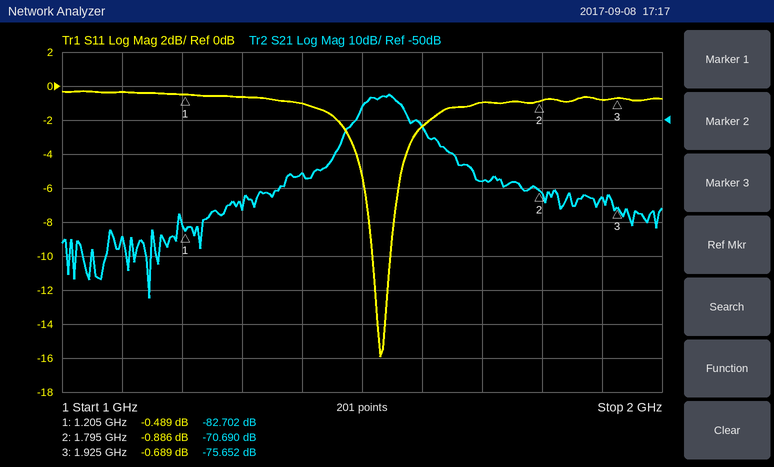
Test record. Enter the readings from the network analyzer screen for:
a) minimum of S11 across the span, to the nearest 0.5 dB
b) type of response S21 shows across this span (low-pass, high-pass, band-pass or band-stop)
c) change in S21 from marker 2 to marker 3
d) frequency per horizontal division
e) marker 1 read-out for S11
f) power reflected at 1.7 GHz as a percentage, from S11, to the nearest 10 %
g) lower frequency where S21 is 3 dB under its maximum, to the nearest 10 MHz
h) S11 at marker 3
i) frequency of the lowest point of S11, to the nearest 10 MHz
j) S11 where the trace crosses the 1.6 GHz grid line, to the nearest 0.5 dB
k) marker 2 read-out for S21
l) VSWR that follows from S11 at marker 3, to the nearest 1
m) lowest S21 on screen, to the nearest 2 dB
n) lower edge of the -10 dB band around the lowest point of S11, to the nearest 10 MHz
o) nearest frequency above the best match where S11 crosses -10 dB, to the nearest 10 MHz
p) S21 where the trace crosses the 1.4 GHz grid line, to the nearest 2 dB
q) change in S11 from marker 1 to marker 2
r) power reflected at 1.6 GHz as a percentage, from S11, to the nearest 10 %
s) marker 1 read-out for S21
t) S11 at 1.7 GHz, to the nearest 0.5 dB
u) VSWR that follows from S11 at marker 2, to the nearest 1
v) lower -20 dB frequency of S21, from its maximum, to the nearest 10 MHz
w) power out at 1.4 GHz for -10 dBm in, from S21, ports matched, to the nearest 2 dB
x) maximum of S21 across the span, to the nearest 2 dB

-16.0 dB
band-pass
-4.962 dB
100 MHz
-0.489 dB
80 %
1.50 GHz
-0.689 dB
1.53 GHz
-2.5 dB
-70.690 dB
25
-102 dB
1.52 GHz
1.55 GHz
-66 dB
-0.397 dB
60 %
-82.702 dB
-1.0 dB
20
1.45 GHz
-76 dBm
-42 dB
